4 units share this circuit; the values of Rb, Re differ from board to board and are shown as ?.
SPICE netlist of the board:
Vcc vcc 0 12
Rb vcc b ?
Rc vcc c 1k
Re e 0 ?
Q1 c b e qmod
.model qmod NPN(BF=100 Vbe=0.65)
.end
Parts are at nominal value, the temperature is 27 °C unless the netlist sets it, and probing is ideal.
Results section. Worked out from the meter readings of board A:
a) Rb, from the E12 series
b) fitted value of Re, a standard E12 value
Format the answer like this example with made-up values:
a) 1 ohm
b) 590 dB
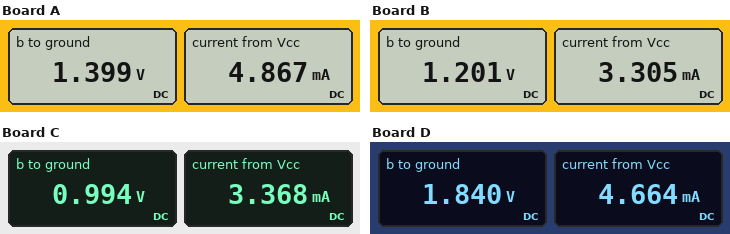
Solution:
a) 220 kΩ
b) 120 Ω
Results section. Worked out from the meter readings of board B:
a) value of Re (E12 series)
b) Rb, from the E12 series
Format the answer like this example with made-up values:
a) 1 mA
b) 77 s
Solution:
a) 120 Ω
b) 330 kΩ
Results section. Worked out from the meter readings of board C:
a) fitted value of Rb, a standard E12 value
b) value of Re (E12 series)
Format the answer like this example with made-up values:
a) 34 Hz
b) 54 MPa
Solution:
a) 330 kΩ
b) 56 Ω
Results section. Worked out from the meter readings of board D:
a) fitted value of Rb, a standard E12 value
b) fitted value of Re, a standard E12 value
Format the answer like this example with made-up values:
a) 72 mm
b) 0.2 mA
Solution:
a) 220 kΩ
b) 220 Ω
